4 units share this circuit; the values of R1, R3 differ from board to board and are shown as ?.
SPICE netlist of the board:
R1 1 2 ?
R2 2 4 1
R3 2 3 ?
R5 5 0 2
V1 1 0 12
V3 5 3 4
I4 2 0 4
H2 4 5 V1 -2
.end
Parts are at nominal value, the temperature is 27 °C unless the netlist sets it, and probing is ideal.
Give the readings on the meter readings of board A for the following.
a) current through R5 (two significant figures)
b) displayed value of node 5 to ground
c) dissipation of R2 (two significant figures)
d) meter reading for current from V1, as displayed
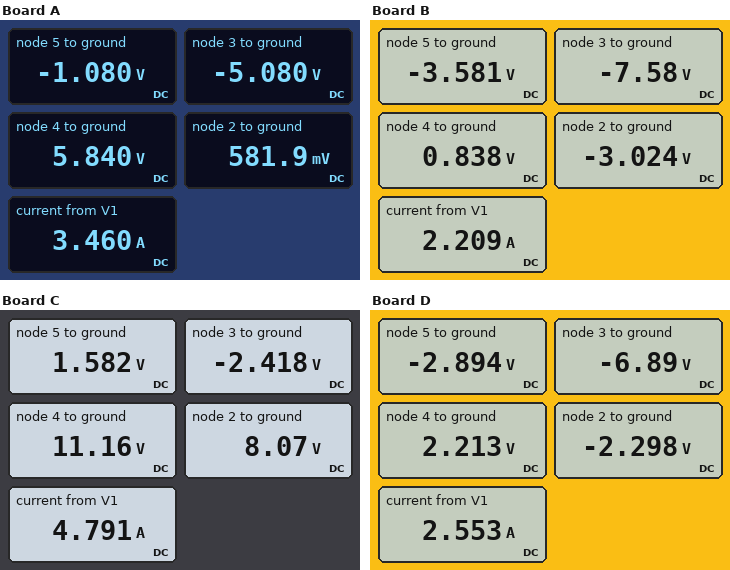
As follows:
540 mA
-1.080 V
28 W
3.460 A
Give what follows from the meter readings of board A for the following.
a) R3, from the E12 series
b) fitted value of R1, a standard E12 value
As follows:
1.2 Ω
3.3 Ω
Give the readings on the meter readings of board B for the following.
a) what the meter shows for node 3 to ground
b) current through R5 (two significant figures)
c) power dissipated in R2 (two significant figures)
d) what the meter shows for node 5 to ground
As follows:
-7.58 V
1.8 A
15 W
-3.581 V
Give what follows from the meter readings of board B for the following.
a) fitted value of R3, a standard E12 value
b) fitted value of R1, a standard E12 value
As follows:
2.2 Ω
6.8 Ω
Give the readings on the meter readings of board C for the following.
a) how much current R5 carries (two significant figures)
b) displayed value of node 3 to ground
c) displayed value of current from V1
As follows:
790 mA
-2.418 V
4.791 A
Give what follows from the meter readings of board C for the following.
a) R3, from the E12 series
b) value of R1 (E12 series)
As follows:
2.7 Ω
0.82 Ω
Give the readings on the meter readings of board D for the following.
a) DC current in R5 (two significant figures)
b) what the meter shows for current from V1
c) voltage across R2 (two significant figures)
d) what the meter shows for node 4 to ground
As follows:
1.4 A
2.553 A
4.5 V
2.213 V
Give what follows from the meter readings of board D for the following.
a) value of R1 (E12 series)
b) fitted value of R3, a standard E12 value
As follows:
5.6 Ω
1.5 Ω
